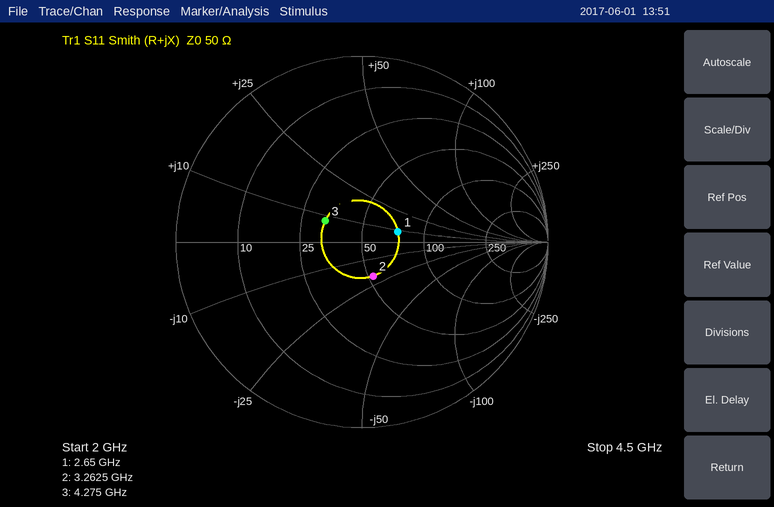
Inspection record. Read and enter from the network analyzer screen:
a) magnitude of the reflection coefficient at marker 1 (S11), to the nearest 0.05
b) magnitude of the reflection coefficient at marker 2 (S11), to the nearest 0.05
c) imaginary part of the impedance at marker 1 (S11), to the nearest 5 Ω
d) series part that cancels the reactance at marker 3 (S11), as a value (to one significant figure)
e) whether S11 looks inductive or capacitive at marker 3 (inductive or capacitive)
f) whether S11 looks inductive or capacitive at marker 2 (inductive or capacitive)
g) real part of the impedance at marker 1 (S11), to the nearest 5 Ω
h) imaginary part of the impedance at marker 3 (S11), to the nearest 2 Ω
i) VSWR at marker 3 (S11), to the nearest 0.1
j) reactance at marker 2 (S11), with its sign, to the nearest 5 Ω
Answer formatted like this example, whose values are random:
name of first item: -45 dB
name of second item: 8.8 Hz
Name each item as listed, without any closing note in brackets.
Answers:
magnitude of the reflection coefficient at marker 1 (S11), to the nearest 0.05: 0.20
magnitude of the reflection coefficient at marker 2 (S11), to the nearest 0.05: 0.20
imaginary part of the impedance at marker 1 (S11), to the nearest 5 Ω: +10 Ω
series part that cancels the reactance at marker 3 (S11), as a value: 5 pF
whether S11 looks inductive or capacitive at marker 3: inductive
whether S11 looks inductive or capacitive at marker 2: capacitive
real part of the impedance at marker 1 (S11), to the nearest 5 Ω: 75 Ω
imaginary part of the impedance at marker 3 (S11), to the nearest 2 Ω: +8 Ω
VSWR at marker 3 (S11), to the nearest 0.1: 1.6
reactance at marker 2 (S11), with its sign, to the nearest 5 Ω: -20 Ω
